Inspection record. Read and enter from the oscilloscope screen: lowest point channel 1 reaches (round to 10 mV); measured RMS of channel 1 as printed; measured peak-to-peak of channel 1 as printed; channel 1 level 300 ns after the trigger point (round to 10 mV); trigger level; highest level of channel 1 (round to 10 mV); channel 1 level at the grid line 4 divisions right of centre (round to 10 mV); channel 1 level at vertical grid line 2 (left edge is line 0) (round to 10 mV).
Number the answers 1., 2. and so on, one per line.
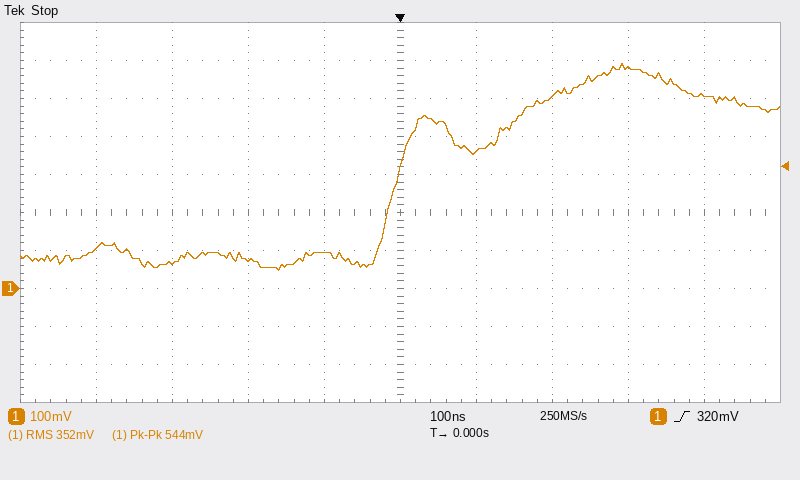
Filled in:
1. 50 mV
2. 352 mV
3. 544 mV
4. 580 mV
5. 320 mV
6. 590 mV
7. 510 mV
8. 70 mV
